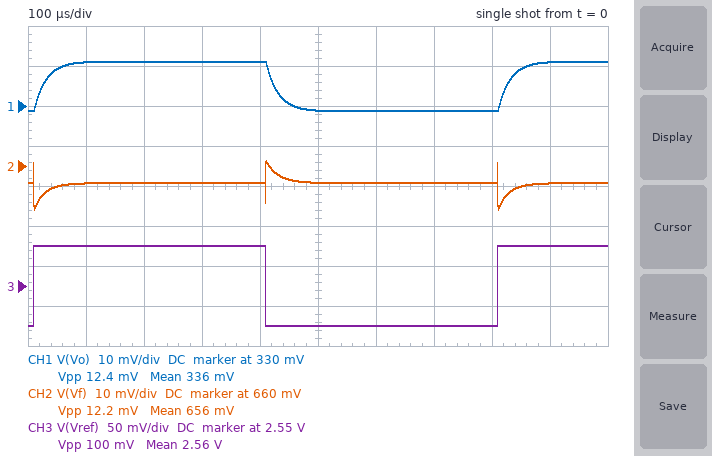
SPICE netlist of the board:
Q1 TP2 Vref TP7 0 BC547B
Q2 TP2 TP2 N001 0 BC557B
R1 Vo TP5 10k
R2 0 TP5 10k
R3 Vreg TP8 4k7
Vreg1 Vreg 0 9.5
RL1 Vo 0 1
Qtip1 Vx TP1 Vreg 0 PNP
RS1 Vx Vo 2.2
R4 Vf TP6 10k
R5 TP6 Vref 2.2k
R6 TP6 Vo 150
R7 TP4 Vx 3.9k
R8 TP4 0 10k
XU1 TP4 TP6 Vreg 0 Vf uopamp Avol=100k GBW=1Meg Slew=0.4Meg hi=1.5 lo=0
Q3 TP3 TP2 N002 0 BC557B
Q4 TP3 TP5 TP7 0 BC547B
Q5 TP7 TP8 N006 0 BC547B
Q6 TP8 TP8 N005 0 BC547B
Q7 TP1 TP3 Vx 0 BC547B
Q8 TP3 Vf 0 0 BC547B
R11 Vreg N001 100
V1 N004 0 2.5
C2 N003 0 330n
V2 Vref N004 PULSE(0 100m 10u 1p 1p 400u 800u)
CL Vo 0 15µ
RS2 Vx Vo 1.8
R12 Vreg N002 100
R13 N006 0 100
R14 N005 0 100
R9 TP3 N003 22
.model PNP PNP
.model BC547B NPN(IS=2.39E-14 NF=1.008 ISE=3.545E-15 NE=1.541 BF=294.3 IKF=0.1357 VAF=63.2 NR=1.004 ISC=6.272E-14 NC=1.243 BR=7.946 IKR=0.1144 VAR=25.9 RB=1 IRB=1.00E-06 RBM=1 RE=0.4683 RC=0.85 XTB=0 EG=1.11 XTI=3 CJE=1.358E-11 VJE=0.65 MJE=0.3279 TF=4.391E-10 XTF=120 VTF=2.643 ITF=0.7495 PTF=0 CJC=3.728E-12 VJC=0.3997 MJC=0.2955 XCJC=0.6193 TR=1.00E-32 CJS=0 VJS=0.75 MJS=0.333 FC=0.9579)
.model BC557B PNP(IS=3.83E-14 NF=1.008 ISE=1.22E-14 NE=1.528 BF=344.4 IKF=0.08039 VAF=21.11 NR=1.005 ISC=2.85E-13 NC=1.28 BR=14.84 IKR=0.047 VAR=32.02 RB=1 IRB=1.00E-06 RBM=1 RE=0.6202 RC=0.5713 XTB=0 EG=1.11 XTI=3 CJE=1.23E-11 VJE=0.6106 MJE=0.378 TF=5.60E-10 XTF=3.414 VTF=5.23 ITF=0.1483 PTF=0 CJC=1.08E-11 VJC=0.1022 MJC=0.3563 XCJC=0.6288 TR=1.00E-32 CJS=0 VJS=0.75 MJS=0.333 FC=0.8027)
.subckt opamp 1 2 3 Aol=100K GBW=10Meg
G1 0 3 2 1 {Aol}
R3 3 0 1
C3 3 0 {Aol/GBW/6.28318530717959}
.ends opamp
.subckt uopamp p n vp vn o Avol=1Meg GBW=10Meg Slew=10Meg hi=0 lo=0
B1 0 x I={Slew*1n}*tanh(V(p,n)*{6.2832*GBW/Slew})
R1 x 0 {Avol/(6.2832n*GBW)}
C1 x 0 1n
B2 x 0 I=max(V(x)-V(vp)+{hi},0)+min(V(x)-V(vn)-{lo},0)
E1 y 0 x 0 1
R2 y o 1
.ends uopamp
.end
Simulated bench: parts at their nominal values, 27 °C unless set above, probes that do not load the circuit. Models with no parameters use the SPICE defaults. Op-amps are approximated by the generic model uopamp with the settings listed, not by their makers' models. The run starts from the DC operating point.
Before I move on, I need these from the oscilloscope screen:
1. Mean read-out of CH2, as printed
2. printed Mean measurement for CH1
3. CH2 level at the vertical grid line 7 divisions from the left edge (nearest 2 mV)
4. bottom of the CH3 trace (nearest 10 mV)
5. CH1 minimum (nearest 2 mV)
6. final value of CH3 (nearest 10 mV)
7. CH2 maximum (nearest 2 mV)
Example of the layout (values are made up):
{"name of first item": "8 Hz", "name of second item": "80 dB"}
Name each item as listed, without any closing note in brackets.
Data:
{"Mean read-out of CH2, as printed": "656 mV", "printed Mean measurement for CH1": "336 mV", "CH2 level at the vertical grid line 7 divisions from the left edge": "656 mV", "bottom of the CH3 trace": "2.50 V", "CH1 minimum": "328 mV", "final value of CH3": "2.60 V", "CH2 maximum": "662 mV"}
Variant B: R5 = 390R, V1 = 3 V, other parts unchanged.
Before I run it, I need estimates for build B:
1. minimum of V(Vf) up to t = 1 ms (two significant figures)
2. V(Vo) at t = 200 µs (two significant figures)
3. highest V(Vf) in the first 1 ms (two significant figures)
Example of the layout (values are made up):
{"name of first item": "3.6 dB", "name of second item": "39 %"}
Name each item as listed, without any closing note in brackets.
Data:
{"minimum of V(Vf) up to t = 1 ms": "600 mV", "V(Vo) at t = 200 µs": "1.2 V", "highest V(Vf) in the first 1 ms": "670 mV"}
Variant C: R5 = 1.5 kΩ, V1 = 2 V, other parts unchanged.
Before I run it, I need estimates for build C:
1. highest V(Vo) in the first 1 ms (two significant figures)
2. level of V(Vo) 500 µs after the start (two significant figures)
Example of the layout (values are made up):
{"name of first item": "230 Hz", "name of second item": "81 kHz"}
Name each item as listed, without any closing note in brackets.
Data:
{"highest V(Vo) in the first 1 ms": "370 mV", "level of V(Vo) 500 µs after the start": "350 mV"}
